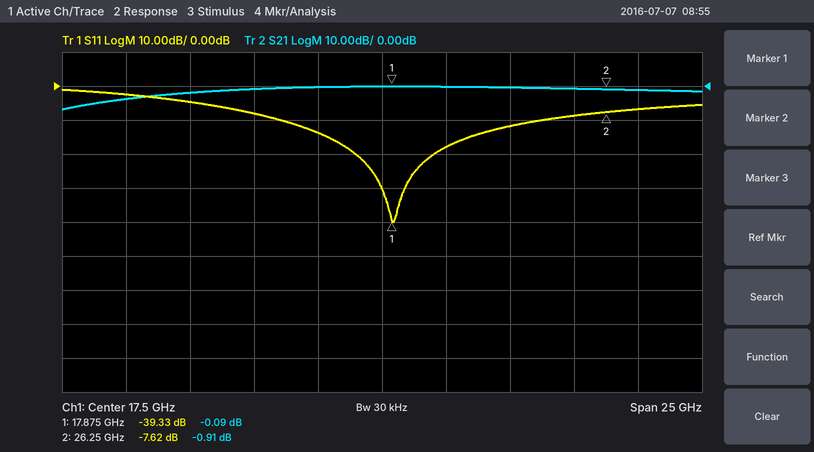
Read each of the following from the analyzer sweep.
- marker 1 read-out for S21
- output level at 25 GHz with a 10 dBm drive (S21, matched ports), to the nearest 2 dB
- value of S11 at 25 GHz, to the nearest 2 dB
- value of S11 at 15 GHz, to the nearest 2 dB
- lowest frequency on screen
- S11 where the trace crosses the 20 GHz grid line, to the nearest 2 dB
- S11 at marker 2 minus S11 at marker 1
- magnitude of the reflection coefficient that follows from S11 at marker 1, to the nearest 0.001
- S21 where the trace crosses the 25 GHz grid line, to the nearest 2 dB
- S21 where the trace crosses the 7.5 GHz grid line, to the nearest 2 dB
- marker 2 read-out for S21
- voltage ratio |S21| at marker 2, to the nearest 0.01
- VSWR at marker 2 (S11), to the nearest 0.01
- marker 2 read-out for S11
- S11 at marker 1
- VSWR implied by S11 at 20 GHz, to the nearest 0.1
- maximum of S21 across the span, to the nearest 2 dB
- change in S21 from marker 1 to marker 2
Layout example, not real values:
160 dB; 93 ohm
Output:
-0.09 dB; 10 dBm; -8 dB; -14 dB; 5 GHz; -18 dB; 31.71 dB; 0.011; 0 dB; -4 dB; -0.91 dB; 0.90; 2.42; -7.62 dB; -39.33 dB; 1.3; 0 dB; -0.82 dB
